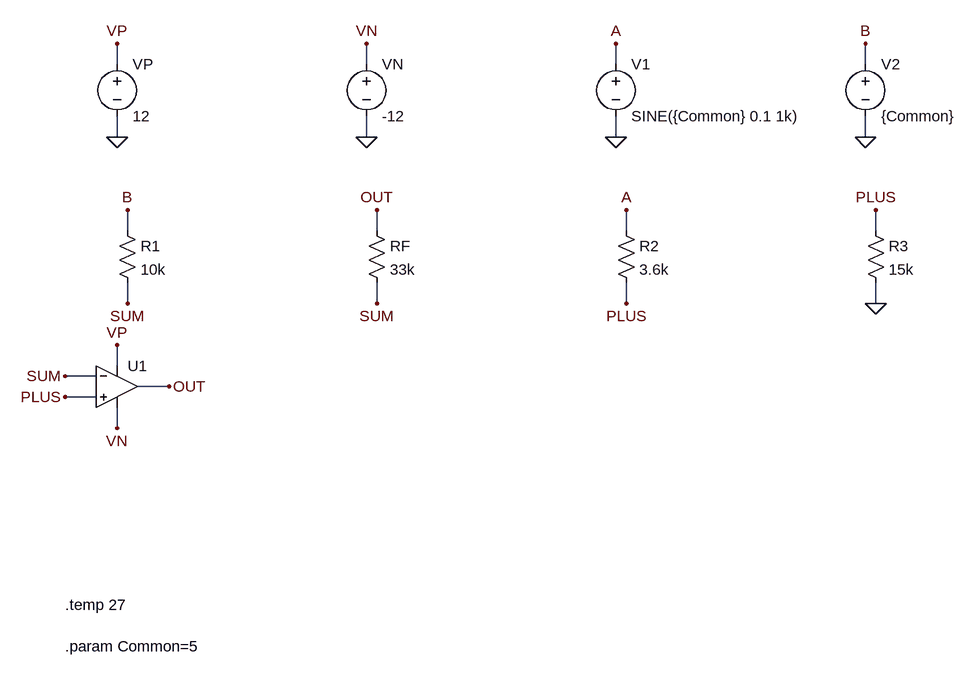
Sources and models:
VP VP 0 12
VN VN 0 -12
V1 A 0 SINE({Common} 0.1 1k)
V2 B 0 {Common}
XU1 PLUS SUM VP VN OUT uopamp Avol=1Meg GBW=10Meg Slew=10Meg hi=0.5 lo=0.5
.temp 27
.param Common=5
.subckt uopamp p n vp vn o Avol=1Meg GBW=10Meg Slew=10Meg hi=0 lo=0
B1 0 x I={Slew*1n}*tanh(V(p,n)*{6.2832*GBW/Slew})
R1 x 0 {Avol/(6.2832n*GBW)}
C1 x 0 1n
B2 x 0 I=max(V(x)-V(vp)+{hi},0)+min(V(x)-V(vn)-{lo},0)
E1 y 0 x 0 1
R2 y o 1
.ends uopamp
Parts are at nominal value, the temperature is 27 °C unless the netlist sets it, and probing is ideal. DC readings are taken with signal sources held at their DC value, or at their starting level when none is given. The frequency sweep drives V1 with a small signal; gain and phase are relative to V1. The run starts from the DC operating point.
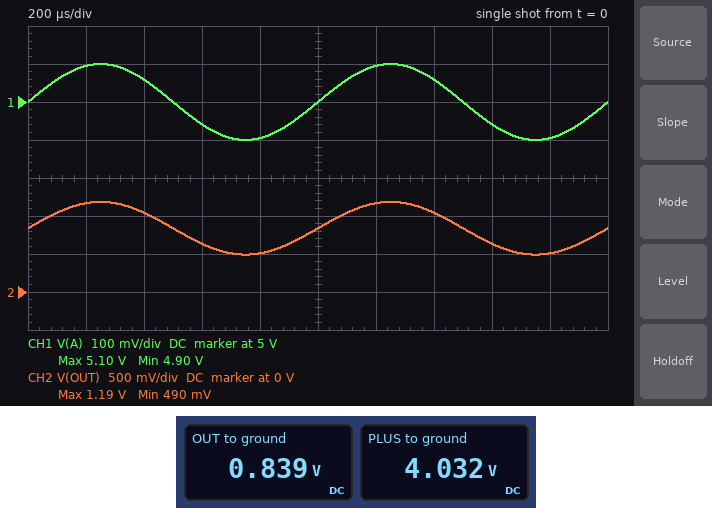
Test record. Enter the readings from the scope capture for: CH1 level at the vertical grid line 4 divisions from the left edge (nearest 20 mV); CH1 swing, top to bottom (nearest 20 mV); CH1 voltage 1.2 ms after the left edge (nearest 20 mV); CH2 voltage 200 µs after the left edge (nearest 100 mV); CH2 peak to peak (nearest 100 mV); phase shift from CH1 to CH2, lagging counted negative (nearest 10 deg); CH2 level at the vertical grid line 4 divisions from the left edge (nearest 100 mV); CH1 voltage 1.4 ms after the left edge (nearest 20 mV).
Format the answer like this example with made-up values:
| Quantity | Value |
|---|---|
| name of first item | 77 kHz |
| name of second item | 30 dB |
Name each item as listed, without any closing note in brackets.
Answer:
| Quantity | Value |
|---|---|
| CH1 level at the vertical grid line 4 divisions from the left edge | 4.90 V |
| CH1 swing, top to bottom | 200 mV |
| CH1 voltage 1.2 ms after the left edge | 5.10 V |
| CH2 voltage 200 µs after the left edge | 1.2 V |
| CH2 peak to peak | 700 mV |
| phase shift from CH1 to CH2, lagging counted negative | 0 deg |
| CH2 level at the vertical grid line 4 divisions from the left edge | 500 mV |
| CH1 voltage 1.4 ms after the left edge | 5.06 V |
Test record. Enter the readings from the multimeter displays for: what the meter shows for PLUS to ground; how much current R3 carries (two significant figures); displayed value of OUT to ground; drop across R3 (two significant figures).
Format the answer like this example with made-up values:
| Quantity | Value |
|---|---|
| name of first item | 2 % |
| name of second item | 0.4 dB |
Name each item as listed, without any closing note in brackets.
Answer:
| Quantity | Value |
|---|---|
| what the meter shows for PLUS to ground | 4.032 V |
| how much current R3 carries | 270 µA |
| displayed value of OUT to ground | 0.839 V |
| drop across R3 | 4.0 V |
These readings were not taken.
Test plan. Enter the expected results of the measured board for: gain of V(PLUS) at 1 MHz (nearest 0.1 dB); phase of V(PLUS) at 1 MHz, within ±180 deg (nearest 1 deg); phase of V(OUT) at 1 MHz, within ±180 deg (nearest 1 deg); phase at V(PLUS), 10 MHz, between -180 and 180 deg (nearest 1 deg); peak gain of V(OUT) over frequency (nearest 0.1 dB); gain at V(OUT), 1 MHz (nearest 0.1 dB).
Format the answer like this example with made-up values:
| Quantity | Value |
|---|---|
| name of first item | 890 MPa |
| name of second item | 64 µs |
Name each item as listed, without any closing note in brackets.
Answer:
| Quantity | Value |
|---|---|
| gain of V(PLUS) at 1 MHz | -1.9 dB |
| phase of V(PLUS) at 1 MHz, within ±180 deg | 0 deg |
| phase of V(OUT) at 1 MHz, within ±180 deg | -23 deg |
| phase at V(PLUS), 10 MHz, between -180 and 180 deg | 0 deg |
| peak gain of V(OUT) over frequency | 10.8 dB |
| gain at V(OUT), 1 MHz | 10.1 dB |
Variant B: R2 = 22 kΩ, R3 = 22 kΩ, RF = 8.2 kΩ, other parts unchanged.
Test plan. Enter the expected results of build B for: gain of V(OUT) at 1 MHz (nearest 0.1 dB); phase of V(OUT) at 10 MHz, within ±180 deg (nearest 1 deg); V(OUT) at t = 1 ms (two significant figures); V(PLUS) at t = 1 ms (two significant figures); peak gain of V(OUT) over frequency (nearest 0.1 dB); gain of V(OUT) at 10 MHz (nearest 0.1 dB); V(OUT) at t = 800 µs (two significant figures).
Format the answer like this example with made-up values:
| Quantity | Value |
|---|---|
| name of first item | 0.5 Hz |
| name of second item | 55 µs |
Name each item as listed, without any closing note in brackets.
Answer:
| Quantity | Value |
|---|---|
| gain of V(OUT) at 1 MHz | -1.0 dB |
| phase of V(OUT) at 10 MHz, within ±180 deg | -61 deg |
| V(OUT) at t = 1 ms | 450 mV |
| V(PLUS) at t = 1 ms | 2.5 V |
| peak gain of V(OUT) over frequency | -0.8 dB |
| gain of V(OUT) at 10 MHz | -7.2 dB |
| V(OUT) at t = 800 µs | 360 mV |
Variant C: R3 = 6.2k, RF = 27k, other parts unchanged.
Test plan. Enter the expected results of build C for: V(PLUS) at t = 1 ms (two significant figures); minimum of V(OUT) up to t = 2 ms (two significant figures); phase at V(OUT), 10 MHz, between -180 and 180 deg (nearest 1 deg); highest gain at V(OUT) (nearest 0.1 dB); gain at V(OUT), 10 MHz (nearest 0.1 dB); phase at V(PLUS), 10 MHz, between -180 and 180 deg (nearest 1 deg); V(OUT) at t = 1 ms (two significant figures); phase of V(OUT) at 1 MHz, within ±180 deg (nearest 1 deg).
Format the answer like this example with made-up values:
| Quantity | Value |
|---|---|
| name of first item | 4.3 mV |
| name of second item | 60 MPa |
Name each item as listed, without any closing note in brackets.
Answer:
| Quantity | Value |
|---|---|
| V(PLUS) at t = 1 ms | 3.2 V |
| minimum of V(OUT) up to t = 2 ms | -2.0 V |
| phase at V(OUT), 10 MHz, between -180 and 180 deg | -75 deg |
| highest gain at V(OUT) | 7.4 dB |
| gain at V(OUT), 10 MHz | -4.3 dB |
| phase at V(PLUS), 10 MHz, between -180 and 180 deg | 0 deg |
| V(OUT) at t = 1 ms | -1.8 V |
| phase of V(OUT) at 1 MHz, within ±180 deg | -20 deg |
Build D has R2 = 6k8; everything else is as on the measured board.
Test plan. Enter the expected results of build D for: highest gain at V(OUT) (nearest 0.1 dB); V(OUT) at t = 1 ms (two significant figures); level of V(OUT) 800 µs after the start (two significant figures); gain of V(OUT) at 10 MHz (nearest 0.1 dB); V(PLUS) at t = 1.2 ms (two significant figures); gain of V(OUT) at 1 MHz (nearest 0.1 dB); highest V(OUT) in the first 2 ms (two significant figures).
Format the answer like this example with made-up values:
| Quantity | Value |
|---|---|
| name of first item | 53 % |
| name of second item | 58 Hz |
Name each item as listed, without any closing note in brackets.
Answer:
| Quantity | Value |
|---|---|
| highest gain at V(OUT) | 9.4 dB |
| V(OUT) at t = 1 ms | -1.7 V |
| level of V(OUT) 800 µs after the start | -2.0 V |
| gain of V(OUT) at 10 MHz | -3.5 dB |
| V(PLUS) at t = 1.2 ms | 3.5 V |
| gain of V(OUT) at 1 MHz | 8.7 dB |
| highest V(OUT) in the first 2 ms | -1.4 V |
